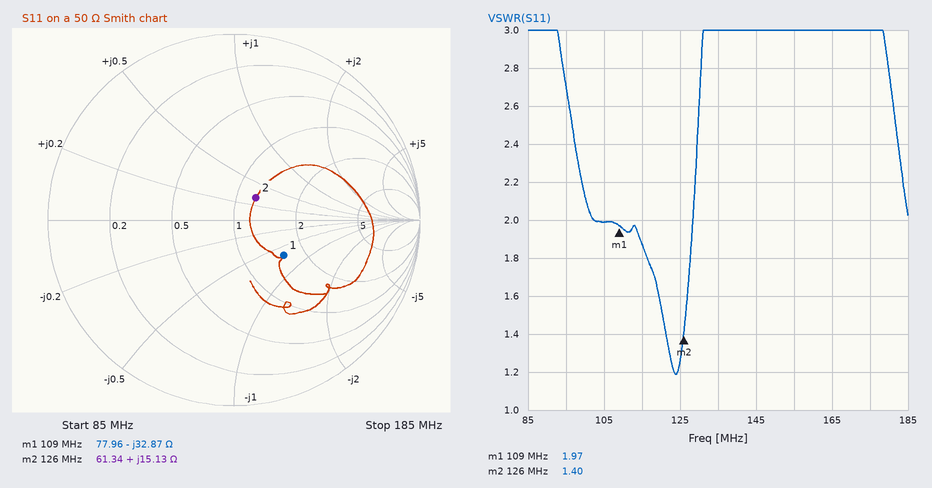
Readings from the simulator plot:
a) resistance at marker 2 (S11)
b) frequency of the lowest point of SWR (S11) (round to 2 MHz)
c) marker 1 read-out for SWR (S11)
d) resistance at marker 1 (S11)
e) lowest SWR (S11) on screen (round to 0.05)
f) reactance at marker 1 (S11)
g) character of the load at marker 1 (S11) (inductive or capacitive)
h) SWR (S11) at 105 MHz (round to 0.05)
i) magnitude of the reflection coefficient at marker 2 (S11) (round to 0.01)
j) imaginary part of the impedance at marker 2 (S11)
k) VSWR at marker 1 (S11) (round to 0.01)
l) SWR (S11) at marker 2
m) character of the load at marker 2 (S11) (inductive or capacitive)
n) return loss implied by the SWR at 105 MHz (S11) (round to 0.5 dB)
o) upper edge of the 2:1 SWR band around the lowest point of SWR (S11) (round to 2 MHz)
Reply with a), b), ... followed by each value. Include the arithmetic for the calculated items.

a) 61.34 Ω
b) 124 MHz
c) 1.97
d) 77.96 Ω
e) 1.20
f) -32.87 Ω
g) capacitive
h) 2.00
i) 0.17
j) +15.13 Ω
k) 1.97
l) 1.40
m) inductive
n) −20 log10((2 − 1)/(2 + 1)) ≈ 9.5 dB
o) 128 MHz
